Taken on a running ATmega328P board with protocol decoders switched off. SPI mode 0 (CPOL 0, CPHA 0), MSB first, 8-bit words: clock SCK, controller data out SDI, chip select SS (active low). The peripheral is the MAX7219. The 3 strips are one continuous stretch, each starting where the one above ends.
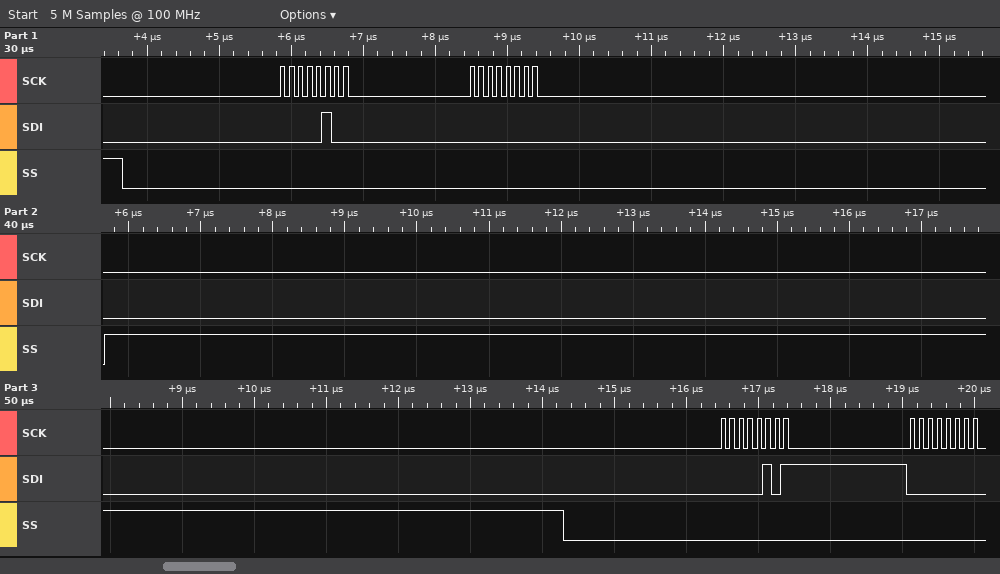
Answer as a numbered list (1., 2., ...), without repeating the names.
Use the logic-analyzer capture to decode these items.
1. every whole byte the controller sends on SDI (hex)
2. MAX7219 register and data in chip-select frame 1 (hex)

1. 04 00 05 00
2. register 0x4, data 0x00
